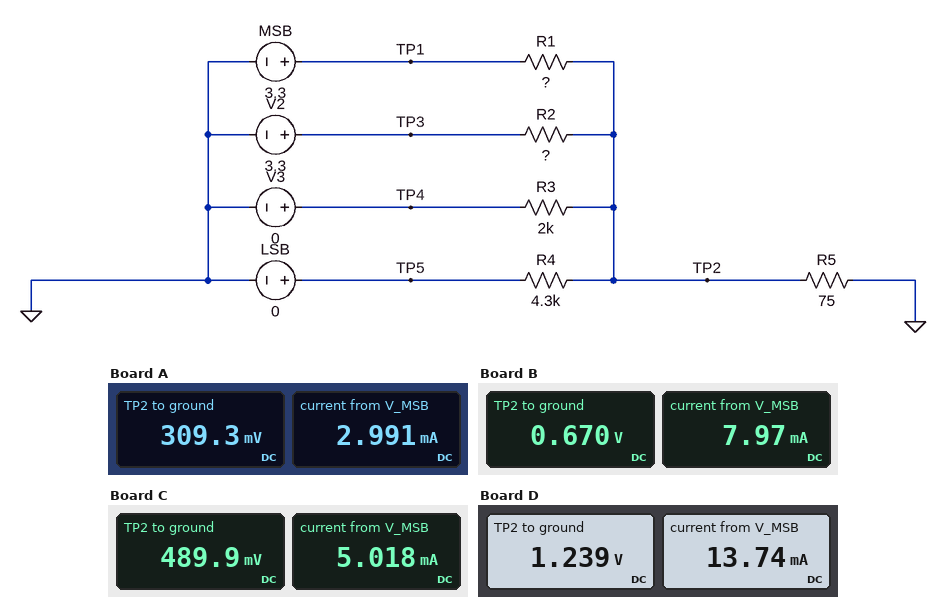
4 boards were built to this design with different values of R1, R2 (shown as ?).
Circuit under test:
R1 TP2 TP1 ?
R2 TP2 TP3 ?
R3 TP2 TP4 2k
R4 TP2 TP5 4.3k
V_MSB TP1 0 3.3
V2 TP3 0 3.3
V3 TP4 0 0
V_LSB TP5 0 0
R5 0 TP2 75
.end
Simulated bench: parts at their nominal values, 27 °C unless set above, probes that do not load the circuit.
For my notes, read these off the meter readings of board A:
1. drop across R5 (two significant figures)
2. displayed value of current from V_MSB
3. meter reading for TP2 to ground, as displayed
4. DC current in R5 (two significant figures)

310 mV
2.991 mA
309.3 mV
4.1 mA
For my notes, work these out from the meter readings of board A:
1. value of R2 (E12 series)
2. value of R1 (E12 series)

2.2 kΩ
1 kΩ
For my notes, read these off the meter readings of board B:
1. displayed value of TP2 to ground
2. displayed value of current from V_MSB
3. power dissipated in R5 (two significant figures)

0.670 V
7.97 mA
6.0 mW
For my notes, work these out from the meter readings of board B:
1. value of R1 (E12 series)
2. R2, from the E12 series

330 Ω
1.8 kΩ
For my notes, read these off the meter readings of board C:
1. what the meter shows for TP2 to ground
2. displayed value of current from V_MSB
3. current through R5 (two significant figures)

489.9 mV
5.018 mA
6.5 mA
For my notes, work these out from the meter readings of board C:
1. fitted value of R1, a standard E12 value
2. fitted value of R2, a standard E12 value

560 Ω
1.5 kΩ
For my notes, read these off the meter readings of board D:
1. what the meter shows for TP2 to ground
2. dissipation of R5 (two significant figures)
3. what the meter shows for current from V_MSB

1.239 V
20 mW
13.74 mA
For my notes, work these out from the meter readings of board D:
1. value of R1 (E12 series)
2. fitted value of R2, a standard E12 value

150 Ω
560 Ω
